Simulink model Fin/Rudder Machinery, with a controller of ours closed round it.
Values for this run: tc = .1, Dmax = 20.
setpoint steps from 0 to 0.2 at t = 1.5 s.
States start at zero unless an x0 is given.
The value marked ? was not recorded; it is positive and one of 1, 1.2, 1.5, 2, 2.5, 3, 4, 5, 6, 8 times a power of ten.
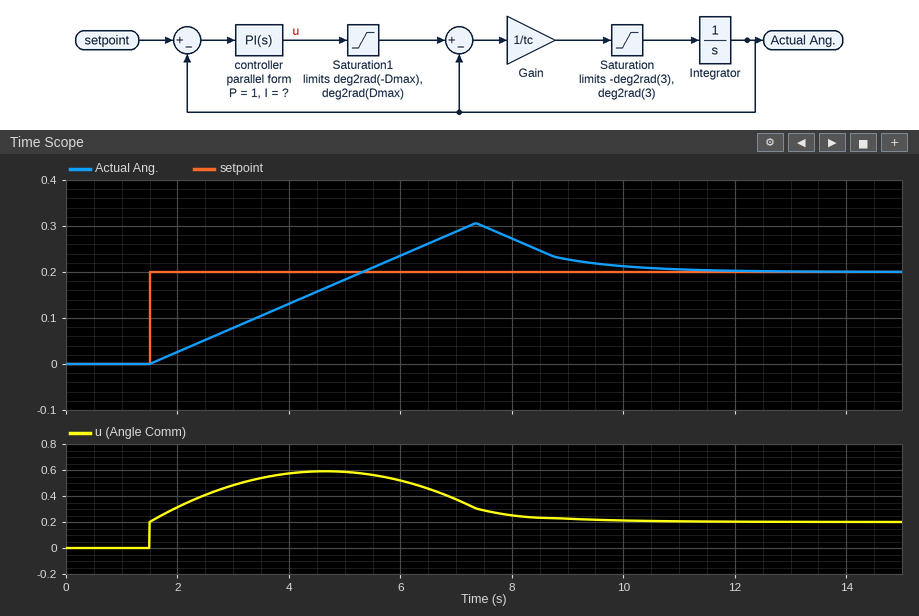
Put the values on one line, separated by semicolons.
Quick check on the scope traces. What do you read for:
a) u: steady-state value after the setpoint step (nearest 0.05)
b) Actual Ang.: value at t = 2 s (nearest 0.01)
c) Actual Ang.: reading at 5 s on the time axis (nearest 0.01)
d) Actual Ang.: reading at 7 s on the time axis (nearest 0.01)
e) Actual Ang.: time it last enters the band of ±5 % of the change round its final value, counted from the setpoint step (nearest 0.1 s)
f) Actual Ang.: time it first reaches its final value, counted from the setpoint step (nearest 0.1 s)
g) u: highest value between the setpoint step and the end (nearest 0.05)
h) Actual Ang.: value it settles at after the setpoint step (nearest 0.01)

0.20; 0.03; 0.18; 0.29; 8.8 s; 3.8 s; 0.60; 0.20
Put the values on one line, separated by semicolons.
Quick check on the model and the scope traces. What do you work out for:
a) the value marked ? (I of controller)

1.5
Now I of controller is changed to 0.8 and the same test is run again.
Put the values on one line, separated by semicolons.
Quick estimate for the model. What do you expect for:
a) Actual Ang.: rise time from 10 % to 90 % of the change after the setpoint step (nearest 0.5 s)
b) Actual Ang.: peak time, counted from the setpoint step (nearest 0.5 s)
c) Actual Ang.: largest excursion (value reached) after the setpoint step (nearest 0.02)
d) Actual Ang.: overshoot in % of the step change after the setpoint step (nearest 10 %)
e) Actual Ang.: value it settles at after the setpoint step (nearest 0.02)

3.0 s; 4.5 s; 0.24; 20 %; 0.20
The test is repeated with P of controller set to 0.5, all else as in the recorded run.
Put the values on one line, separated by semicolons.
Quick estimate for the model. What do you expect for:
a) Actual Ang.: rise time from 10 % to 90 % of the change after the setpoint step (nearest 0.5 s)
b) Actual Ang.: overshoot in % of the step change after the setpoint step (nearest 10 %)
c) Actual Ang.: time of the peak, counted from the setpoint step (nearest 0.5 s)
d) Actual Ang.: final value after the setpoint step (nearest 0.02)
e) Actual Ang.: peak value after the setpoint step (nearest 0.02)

3.0 s; 60 %; 6.0 s; 0.20; 0.32
